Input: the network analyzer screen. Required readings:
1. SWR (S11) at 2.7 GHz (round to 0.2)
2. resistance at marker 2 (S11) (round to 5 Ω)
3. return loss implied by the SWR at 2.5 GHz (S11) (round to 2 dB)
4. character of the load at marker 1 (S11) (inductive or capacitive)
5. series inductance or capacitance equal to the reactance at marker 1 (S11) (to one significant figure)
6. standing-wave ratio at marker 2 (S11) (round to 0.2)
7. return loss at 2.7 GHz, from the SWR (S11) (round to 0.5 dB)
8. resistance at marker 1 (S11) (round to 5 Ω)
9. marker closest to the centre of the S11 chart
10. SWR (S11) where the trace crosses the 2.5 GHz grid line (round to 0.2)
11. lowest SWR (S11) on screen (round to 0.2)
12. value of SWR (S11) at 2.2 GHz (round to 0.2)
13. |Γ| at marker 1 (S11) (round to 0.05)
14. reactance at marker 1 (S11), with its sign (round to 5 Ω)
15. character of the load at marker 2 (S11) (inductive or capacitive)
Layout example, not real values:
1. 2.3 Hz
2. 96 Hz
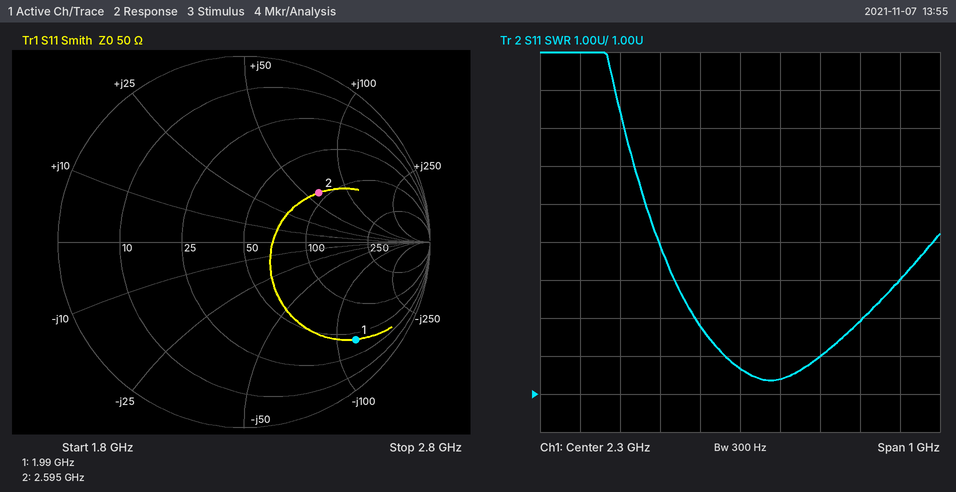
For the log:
1. 4.0
2. 90 Ω
3. 10 dB
4. capacitive
5. 700 fF
6. 2.8
7. 4.5 dB
8. 40 Ω
9. marker 2
10. 2.0
11. 1.4
12. 2.8
13. 0.80
14. -120 Ω
15. inductive
